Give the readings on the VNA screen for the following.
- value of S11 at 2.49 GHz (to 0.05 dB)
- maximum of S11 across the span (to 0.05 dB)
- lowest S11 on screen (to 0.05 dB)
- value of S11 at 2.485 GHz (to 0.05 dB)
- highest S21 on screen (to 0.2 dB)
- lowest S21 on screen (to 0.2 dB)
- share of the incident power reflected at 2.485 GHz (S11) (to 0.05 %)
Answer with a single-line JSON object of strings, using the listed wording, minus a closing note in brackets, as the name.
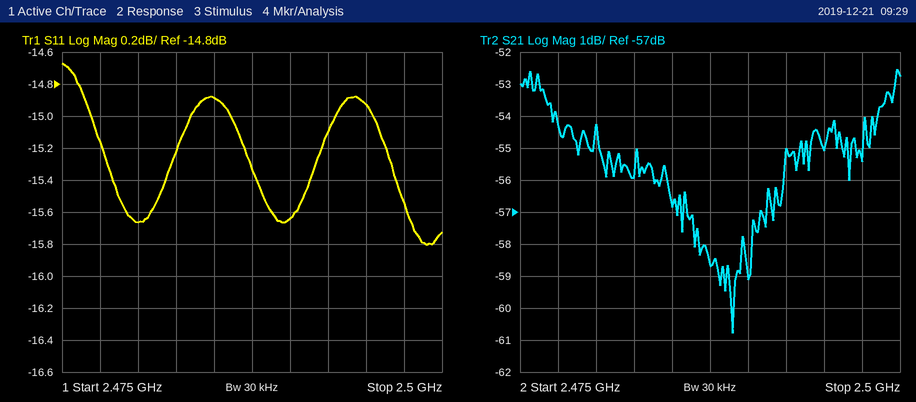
{"value of S11 at 2.49 GHz": "-15.65 dB", "maximum of S11 across the span": "-14.65 dB", "lowest S11 on screen": "-15.80 dB", "value of S11 at 2.485 GHz": "-14.90 dB", "highest S21 on screen": "-52.6 dB", "lowest S21 on screen": "-60.8 dB", "share of the incident power reflected at 2.485 GHz (S11)": "3.25 %"}
